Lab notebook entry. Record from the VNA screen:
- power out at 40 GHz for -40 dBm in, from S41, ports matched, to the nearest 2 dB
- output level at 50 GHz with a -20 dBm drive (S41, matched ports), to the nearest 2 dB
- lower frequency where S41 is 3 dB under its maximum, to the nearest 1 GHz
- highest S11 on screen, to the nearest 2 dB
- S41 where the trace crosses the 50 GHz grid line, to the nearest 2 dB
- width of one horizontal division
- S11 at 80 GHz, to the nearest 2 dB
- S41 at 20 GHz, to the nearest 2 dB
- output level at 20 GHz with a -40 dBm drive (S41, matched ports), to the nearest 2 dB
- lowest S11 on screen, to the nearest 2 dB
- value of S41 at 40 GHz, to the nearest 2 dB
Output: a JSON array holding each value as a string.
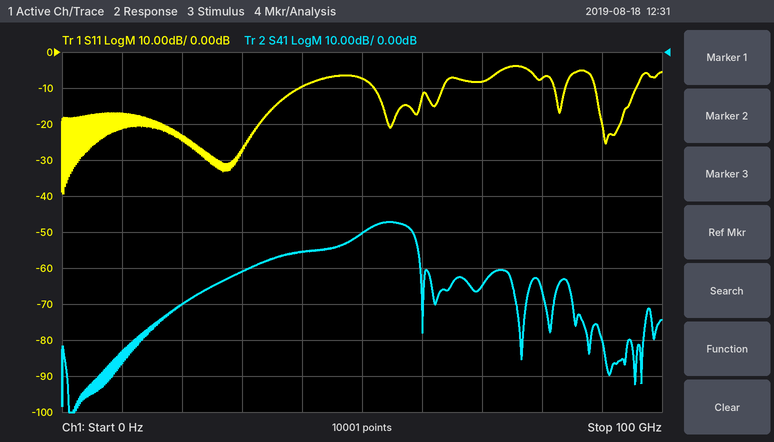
["-96 dBm", "-70 dBm", "50 GHz", "-4 dB", "-50 dB", "10 GHz", "-8 dB", "-70 dB", "-110 dBm", "-40 dB", "-56 dB"]
